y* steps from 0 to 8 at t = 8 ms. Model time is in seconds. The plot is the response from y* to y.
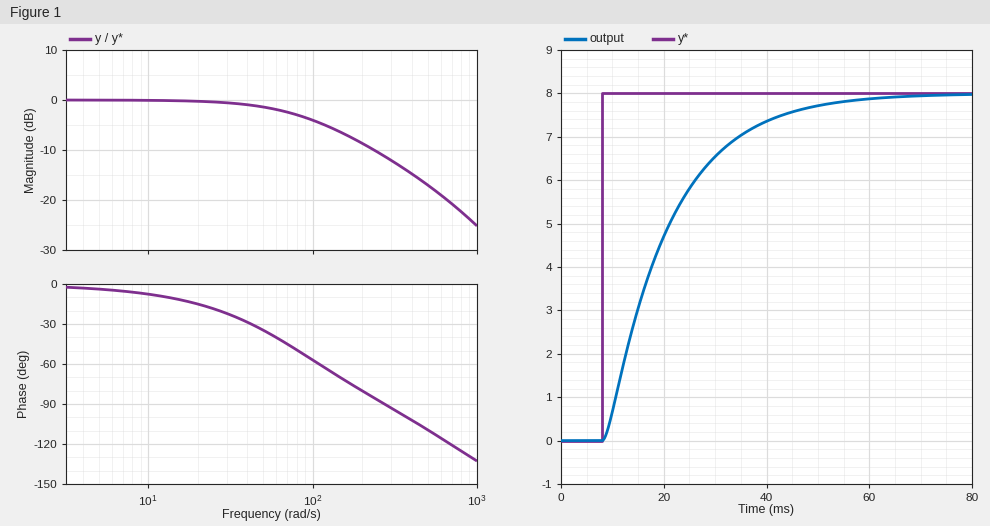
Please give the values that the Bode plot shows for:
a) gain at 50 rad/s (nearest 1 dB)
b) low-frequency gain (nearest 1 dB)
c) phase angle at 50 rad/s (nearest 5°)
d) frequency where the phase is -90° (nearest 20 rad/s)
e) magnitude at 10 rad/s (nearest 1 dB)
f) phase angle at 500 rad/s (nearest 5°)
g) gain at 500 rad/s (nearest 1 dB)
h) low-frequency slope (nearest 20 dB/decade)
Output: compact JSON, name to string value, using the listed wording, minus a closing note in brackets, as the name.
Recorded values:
{"gain at 50 rad/s": "-1 dB", "low-frequency gain": "0 dB", "phase angle at 50 rad/s": "-35°", "frequency where the phase is -90°": "280 rad/s", "magnitude at 10 rad/s": "0 dB", "phase angle at 500 rad/s": "-110°", "gain at 500 rad/s": "-17 dB", "low-frequency slope": "0 dB/decade"}
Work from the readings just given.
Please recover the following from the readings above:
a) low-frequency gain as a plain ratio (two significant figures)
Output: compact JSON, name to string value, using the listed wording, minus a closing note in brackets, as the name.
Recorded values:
{"low-frequency gain as a plain ratio": "1.0"}
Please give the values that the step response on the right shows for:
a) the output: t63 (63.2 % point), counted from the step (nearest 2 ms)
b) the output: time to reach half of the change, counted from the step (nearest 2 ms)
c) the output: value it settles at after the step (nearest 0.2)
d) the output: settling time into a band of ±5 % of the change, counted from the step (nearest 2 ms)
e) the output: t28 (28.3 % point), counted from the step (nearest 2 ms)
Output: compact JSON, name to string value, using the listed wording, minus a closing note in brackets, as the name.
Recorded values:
{"the output: t63 (63.2 % point), counted from the step": "14 ms", "the output: time to reach half of the change, counted from the step": "10 ms", "the output: value it settles at after the step": "8.0", "the output: settling time into a band of ±5 % of the change, counted from the step": "38 ms", "the output: t28 (28.3 % point), counted from the step": "6 ms"}
